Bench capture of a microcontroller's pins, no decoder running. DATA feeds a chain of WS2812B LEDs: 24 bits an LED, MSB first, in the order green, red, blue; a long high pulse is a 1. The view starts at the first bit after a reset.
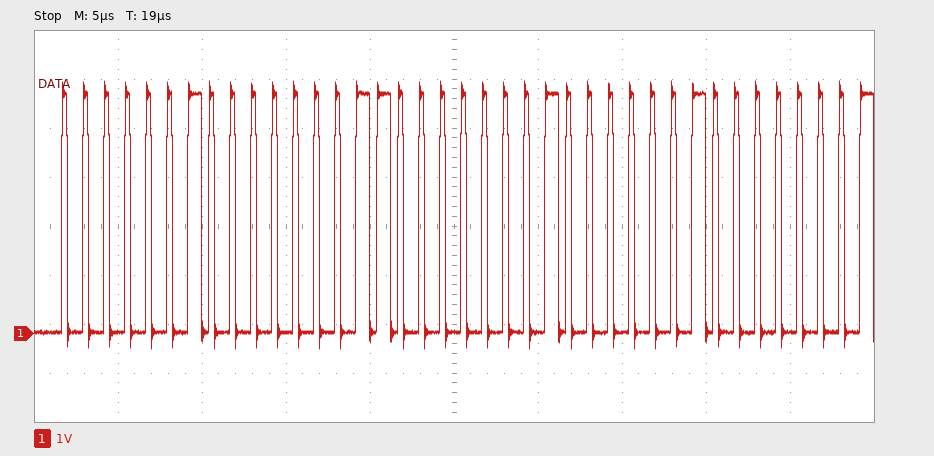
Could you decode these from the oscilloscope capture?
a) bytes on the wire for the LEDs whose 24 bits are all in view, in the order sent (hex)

02 03 01
